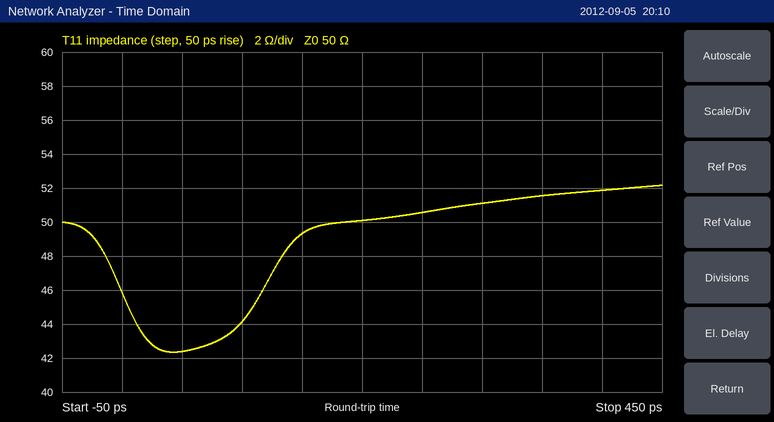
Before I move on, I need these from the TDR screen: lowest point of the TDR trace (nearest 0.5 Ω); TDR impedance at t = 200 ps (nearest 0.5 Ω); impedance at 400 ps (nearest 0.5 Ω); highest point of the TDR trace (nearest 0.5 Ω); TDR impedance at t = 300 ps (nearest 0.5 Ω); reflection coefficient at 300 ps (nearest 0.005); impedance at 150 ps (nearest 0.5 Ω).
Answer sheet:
42.5 Ω
50.0 Ω
52.0 Ω
52.0 Ω
51.0 Ω
+0.010
49.5 Ω
